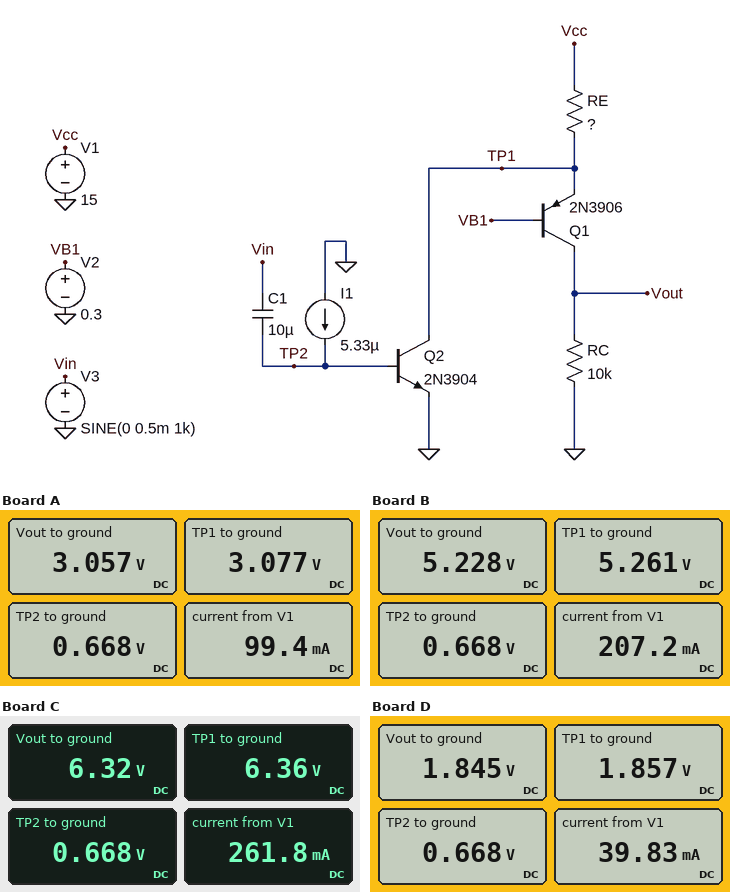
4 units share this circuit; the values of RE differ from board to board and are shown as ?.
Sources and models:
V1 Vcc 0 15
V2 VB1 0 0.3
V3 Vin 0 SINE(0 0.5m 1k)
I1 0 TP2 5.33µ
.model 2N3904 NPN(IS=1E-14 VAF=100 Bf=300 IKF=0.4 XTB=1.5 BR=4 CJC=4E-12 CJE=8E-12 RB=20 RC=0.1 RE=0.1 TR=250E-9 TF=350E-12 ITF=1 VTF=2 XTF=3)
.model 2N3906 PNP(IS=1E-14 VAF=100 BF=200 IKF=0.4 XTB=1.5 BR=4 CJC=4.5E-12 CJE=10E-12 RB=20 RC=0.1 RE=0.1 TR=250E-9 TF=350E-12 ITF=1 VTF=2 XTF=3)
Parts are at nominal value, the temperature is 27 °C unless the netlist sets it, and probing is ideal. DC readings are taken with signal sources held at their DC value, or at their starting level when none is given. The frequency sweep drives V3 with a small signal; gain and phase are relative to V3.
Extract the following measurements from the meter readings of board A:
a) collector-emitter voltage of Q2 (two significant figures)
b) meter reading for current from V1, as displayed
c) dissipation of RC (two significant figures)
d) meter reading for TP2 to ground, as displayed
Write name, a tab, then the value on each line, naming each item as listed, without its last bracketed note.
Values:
collector-emitter voltage of Q2	3.1 V
meter reading for current from V1, as displayed	99.4 mA
dissipation of RC	930 µW
meter reading for TP2 to ground, as displayed	0.668 V
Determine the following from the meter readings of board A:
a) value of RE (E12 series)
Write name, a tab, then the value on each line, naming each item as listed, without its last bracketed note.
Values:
value of RE	120 Ω
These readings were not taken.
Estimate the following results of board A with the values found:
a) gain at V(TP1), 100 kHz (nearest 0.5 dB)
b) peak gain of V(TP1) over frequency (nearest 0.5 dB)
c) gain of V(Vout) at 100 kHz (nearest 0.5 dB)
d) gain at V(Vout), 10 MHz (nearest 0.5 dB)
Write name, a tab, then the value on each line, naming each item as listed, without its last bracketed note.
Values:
gain at V(TP1), 100 kHz	0.5 dB
peak gain of V(TP1) over frequency	0.5 dB
gain of V(Vout) at 100 kHz	0.5 dB
gain at V(Vout), 10 MHz	0.5 dB
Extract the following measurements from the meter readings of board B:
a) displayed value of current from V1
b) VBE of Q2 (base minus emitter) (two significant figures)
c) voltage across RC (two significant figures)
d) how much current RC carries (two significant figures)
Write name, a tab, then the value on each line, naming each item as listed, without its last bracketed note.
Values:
displayed value of current from V1	207.2 mA
VBE of Q2 (base minus emitter)	670 mV
voltage across RC	5.2 V
how much current RC carries	520 µA
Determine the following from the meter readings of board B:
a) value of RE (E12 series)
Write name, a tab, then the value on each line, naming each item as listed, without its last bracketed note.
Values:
value of RE	47 Ω
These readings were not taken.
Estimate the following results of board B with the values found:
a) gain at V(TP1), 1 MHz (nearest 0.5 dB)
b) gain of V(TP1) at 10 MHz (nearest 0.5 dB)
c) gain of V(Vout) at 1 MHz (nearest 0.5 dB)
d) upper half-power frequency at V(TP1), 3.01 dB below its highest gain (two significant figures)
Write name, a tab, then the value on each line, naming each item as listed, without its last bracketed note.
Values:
gain at V(TP1), 1 MHz	-1.0 dB
gain of V(TP1) at 10 MHz	-1.0 dB
gain of V(Vout) at 1 MHz	-1.0 dB
upper half-power frequency at V(TP1), 3.01 dB below its highest gain	200 MHz
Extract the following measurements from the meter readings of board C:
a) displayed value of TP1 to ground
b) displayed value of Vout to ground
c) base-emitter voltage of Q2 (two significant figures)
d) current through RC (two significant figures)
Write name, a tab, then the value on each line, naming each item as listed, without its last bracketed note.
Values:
displayed value of TP1 to ground	6.36 V
displayed value of Vout to ground	6.32 V
base-emitter voltage of Q2	670 mV
current through RC	630 µA
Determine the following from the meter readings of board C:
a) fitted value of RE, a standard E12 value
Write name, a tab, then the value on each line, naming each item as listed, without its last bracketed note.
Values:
fitted value of RE, a standard E12 value	33 Ω
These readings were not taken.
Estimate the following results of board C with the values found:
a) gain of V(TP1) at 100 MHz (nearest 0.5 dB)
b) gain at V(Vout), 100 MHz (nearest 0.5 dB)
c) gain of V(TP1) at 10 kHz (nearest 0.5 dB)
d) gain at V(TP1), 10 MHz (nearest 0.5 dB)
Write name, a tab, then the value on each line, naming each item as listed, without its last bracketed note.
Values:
gain of V(TP1) at 100 MHz	-3.0 dB
gain at V(Vout), 100 MHz	-3.0 dB
gain of V(TP1) at 10 kHz	-2.0 dB
gain at V(TP1), 10 MHz	-2.0 dB
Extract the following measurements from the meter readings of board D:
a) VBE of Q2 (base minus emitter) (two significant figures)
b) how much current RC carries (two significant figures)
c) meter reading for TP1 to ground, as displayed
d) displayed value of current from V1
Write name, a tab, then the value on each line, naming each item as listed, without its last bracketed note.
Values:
VBE of Q2 (base minus emitter)	670 mV
how much current RC carries	180 µA
meter reading for TP1 to ground, as displayed	1.857 V
displayed value of current from V1	39.83 mA
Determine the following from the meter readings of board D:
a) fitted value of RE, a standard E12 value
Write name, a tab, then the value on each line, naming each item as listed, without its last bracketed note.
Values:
fitted value of RE, a standard E12 value	330 Ω
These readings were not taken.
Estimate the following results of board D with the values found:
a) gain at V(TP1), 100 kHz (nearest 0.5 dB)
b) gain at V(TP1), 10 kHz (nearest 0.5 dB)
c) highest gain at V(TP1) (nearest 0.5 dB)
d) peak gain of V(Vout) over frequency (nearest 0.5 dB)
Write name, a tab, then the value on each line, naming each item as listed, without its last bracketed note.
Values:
gain at V(TP1), 100 kHz	1.5 dB
gain at V(TP1), 10 kHz	1.5 dB
highest gain at V(TP1)	1.5 dB
peak gain of V(Vout) over frequency	1.5 dB
